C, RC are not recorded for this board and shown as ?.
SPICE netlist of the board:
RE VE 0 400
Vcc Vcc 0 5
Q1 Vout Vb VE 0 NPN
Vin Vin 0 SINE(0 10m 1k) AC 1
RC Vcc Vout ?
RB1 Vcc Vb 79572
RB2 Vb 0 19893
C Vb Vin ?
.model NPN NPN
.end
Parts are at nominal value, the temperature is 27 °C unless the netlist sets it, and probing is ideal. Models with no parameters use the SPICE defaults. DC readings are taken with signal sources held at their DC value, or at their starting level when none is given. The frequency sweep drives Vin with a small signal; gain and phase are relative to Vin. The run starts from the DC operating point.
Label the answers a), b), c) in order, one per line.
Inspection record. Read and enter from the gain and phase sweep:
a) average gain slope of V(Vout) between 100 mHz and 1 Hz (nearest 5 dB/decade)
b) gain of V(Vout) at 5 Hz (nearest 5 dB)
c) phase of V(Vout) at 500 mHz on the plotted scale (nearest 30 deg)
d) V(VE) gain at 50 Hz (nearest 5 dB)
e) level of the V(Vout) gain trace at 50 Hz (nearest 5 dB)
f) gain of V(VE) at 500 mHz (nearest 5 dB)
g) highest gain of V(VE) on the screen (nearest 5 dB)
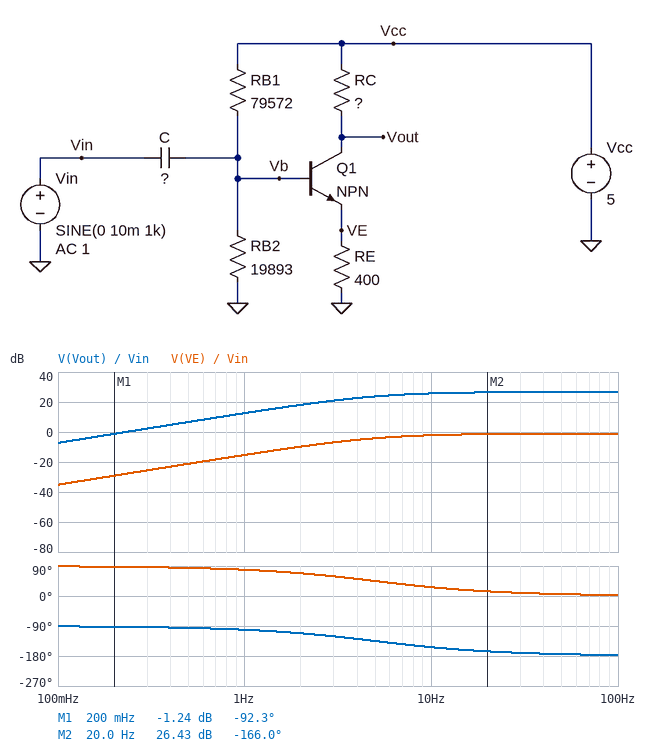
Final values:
a) 20 dB/decade
b) 25 dB
c) -90 deg
d) 0 dB
e) 25 dB
f) -20 dB
g) 0 dB
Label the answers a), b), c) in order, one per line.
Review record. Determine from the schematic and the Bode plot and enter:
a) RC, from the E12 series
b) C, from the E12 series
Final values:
a) 10 kΩ
b) 2.7 µF
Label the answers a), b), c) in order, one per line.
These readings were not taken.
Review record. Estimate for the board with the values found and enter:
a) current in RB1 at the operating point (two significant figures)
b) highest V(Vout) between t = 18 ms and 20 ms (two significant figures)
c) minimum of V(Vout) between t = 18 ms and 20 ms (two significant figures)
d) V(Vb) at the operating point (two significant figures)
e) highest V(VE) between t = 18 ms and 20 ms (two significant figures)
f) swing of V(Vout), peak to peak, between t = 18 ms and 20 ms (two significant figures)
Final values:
a) 51 µA
b) 830 mV
c) 400 mV
d) 930 mV
e) 190 mV
f) 430 mV
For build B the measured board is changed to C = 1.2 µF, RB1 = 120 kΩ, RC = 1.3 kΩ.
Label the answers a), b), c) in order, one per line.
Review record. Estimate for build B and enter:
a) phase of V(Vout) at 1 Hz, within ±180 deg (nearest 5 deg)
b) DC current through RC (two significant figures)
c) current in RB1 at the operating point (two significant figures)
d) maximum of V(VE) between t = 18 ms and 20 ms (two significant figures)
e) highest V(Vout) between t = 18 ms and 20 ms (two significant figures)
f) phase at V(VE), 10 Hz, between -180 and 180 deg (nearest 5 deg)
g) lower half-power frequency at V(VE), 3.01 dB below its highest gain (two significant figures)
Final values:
a) -95 deg
b) 38 µA
c) 36 µA
d) 19 mV
e) 5.0 V
f) 40 deg
g) 9.0 Hz
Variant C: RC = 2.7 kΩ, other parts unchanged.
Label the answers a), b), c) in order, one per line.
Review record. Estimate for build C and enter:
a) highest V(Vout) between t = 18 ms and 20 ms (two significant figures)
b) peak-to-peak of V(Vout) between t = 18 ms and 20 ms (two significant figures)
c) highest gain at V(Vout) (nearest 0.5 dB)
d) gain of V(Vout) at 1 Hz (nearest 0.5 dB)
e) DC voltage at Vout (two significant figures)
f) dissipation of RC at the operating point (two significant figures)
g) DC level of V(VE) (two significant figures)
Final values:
a) 3.9 V
b) 120 mV
c) 15.5 dB
d) 1.0 dB
e) 3.8 V
f) 520 µW
g) 180 mV
